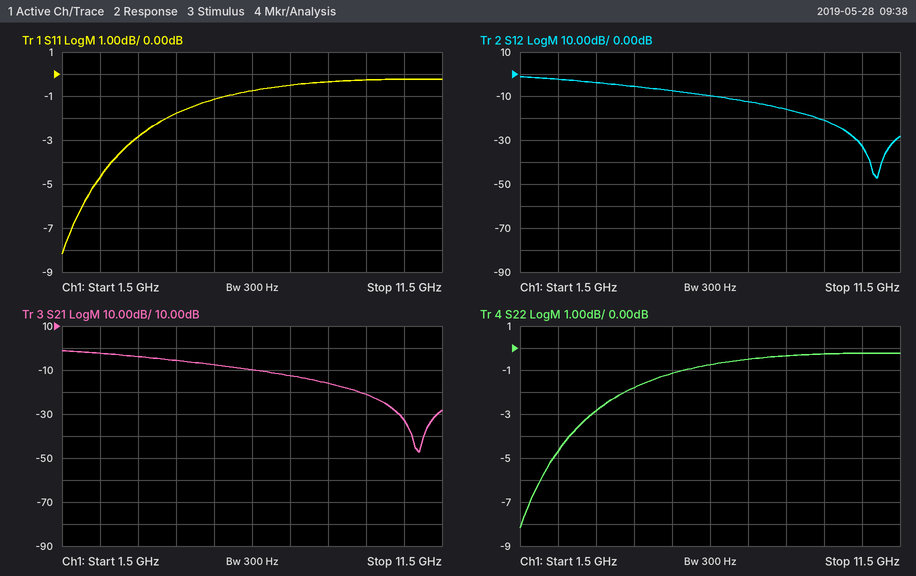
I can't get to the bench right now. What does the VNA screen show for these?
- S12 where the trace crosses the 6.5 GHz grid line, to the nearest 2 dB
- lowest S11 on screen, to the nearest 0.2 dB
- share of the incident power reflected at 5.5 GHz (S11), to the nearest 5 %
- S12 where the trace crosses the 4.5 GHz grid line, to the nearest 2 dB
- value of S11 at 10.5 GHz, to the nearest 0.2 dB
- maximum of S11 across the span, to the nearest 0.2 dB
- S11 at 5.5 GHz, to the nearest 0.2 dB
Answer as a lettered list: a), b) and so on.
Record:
a) -10 dB
b) -8.2 dB
c) 75 %
d) -6 dB
e) -0.2 dB
f) -0.2 dB
g) -1.2 dB
